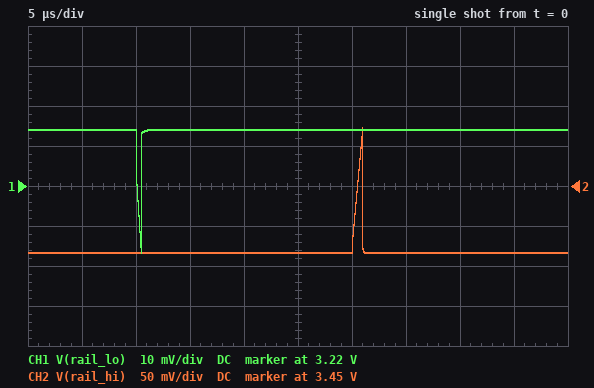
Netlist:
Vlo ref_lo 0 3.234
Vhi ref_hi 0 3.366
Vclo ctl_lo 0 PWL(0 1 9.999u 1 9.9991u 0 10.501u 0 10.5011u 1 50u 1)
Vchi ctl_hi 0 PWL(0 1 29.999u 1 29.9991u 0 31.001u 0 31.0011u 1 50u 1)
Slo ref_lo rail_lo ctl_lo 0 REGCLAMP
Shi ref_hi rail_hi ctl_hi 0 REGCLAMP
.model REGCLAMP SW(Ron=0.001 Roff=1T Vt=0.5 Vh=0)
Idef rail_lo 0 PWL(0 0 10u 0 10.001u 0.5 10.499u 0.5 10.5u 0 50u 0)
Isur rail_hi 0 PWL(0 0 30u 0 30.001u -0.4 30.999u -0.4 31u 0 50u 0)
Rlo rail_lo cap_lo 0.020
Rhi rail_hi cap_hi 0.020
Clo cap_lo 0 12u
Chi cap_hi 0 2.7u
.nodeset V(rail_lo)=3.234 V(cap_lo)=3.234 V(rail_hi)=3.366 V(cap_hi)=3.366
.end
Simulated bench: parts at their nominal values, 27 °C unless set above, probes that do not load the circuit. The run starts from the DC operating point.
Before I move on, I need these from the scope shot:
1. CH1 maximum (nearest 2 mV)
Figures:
3.234 V
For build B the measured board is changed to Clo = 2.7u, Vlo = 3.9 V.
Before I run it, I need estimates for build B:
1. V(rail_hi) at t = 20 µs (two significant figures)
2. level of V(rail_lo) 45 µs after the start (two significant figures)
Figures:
3.4 V
3.9 V
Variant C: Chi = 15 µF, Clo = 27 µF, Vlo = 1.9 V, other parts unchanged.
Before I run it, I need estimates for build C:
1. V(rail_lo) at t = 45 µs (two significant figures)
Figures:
1.9 V
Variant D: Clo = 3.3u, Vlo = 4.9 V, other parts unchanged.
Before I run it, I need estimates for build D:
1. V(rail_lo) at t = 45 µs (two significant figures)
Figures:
4.9 V
